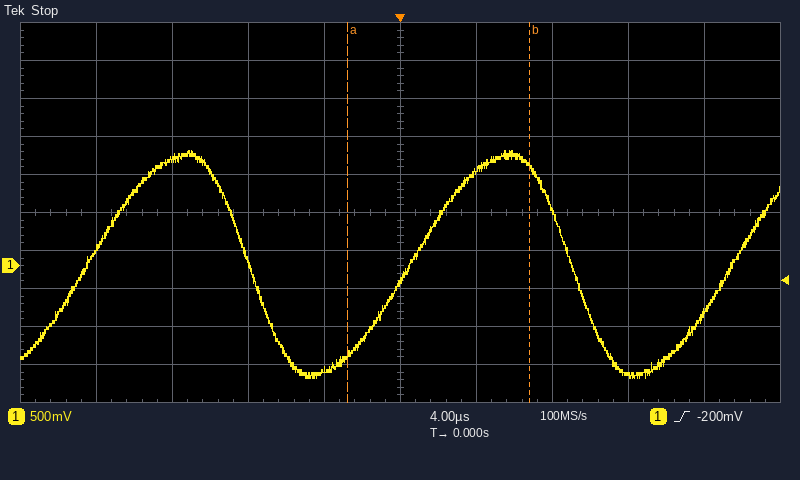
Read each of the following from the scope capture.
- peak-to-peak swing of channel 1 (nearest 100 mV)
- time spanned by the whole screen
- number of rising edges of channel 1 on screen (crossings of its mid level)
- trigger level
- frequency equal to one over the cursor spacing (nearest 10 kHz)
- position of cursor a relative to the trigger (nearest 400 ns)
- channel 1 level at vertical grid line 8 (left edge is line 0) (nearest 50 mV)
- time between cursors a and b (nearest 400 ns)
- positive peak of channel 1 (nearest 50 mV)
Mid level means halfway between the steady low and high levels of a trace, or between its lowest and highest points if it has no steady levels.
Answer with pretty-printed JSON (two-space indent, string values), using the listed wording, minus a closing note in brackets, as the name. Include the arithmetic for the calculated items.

{
  "peak-to-peak swing of channel 1": "3.00 V",
  "time spanned by the whole screen": "40 µs",
  "number of rising edges of channel 1 on screen": "3",
  "trigger level": "-200 mV",
  "frequency equal to one over the cursor spacing": "1 / 9.6 µs ≈ 100 kHz",
  "position of cursor a relative to the trigger": "-2.8 µs",
  "channel 1 level at vertical grid line 8 (left edge is line 0)": "-1.45 V",
  "time between cursors a and b": "9.6 µs",
  "positive peak of channel 1": "1.50 V"
}
